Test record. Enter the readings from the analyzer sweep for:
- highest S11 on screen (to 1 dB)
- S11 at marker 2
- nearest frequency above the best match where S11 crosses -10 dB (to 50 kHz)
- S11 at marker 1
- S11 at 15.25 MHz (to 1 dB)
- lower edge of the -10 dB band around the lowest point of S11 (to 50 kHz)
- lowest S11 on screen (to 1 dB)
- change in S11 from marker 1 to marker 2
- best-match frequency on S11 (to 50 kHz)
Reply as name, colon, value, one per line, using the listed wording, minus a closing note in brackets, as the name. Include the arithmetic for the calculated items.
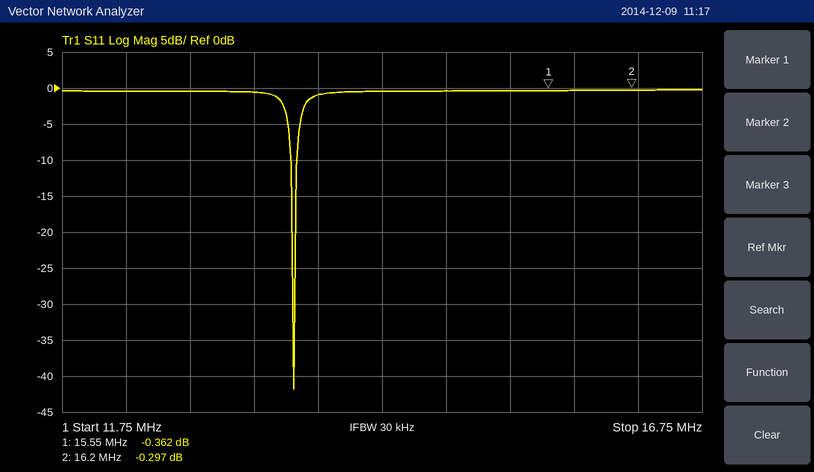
highest S11 on screen: 0 dB
S11 at marker 2: -0.297 dB
nearest frequency above the best match where S11 crosses -10 dB: 13.60 MHz
S11 at marker 1: -0.362 dB
S11 at 15.25 MHz: 0 dB
lower edge of the -10 dB band around the lowest point of S11: 13.55 MHz
lowest S11 on screen: -42 dB
change in S11 from marker 1 to marker 2: -0.297 − (-0.362) = 0.065 dB
best-match frequency on S11: 13.55 MHz
